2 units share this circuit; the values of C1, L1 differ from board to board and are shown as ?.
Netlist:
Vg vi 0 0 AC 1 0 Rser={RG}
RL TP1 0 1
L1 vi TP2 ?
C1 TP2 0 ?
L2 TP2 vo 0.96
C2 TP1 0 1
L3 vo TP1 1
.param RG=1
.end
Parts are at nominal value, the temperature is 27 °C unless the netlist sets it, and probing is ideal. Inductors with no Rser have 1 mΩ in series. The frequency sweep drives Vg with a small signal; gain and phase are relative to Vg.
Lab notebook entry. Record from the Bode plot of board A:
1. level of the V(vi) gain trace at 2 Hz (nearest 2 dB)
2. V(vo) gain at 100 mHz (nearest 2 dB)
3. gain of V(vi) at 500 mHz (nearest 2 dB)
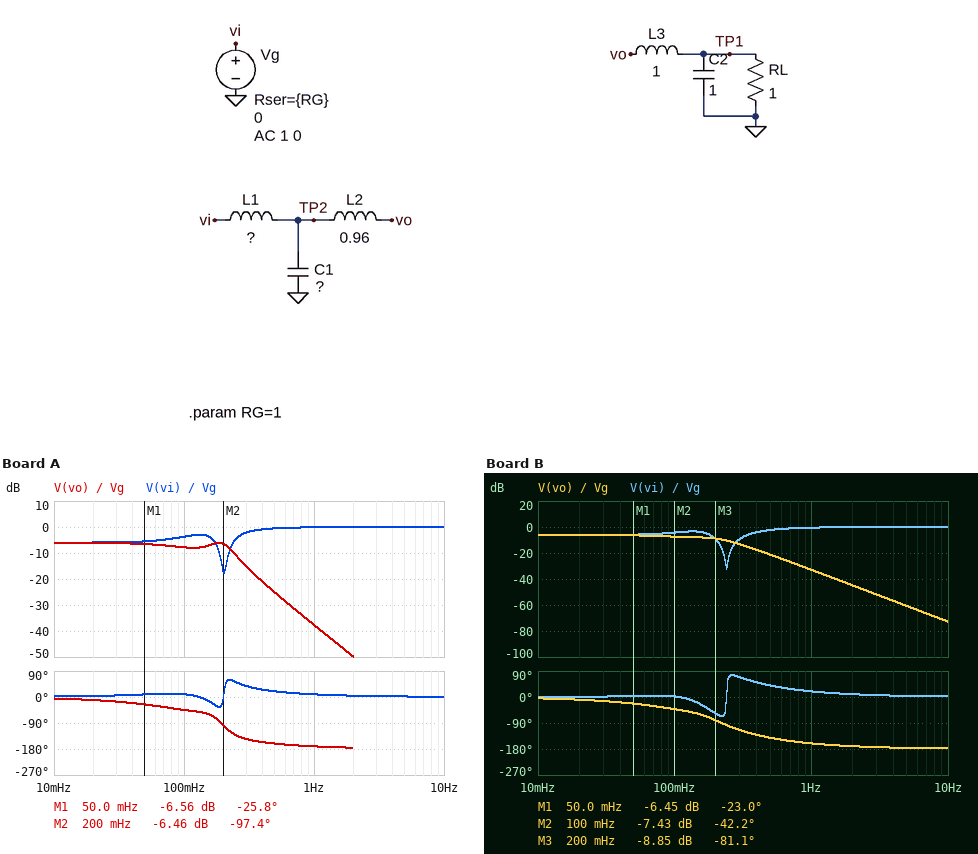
0 dB
-8 dB
0 dB
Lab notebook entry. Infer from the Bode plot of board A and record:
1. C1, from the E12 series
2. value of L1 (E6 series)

1 F
1 H
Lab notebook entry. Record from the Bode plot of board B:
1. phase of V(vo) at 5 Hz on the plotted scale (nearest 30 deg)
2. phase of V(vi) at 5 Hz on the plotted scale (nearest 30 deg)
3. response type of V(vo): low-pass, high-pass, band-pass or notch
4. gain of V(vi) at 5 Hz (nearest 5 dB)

-180 deg
0 deg
low-pass
0 dB
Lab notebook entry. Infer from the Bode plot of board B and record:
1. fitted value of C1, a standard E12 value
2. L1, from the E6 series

1.2 F
470 mH
